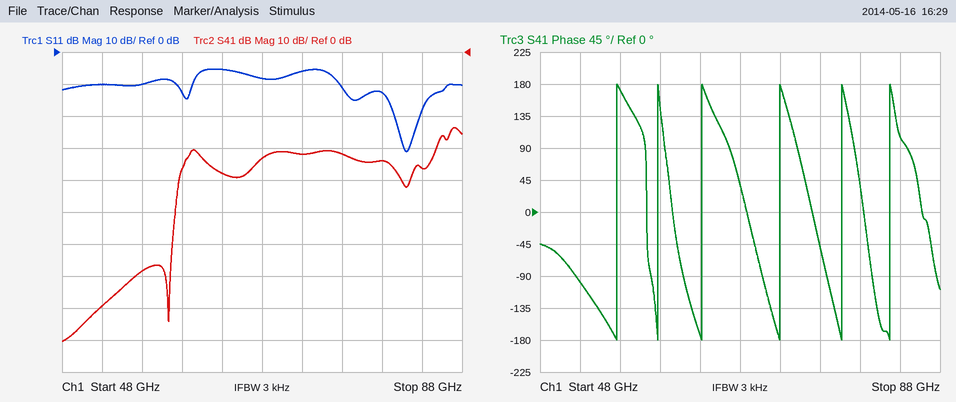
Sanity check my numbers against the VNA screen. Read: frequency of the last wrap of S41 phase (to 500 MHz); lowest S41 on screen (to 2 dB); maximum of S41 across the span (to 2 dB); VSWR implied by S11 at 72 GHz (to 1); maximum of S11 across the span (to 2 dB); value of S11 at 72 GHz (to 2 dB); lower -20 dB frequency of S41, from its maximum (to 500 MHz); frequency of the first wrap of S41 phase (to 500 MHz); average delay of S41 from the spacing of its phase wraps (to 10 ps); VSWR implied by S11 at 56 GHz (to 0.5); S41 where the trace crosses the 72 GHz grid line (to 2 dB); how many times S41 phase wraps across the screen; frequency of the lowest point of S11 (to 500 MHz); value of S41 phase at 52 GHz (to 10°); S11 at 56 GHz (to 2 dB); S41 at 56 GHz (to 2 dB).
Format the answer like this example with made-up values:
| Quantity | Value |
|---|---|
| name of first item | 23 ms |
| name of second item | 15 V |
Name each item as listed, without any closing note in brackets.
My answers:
| Quantity | Value |
|---|---|
| frequency of the last wrap of S41 phase | 83.0 GHz |
| lowest S41 on screen | -90 dB |
| maximum of S41 across the span | -24 dB |
| VSWR implied by S11 at 72 GHz | 3 |
| maximum of S11 across the span | -6 dB |
| value of S11 at 72 GHz | -6 dB |
| lower -20 dB frequency of S41, from its maximum | 59.5 GHz |
| frequency of the first wrap of S41 phase | 55.5 GHz |
| average delay of S41 from the spacing of its phase wraps | 180 ps |
| VSWR implied by S11 at 56 GHz | 2.0 |
| S41 where the trace crosses the 72 GHz grid line | -32 dB |
| how many times S41 phase wraps across the screen | 6 |
| frequency of the lowest point of S11 | 82.5 GHz |
| value of S41 phase at 52 GHz | -100° |
| S11 at 56 GHz | -10 dB |
| S41 at 56 GHz | -68 dB |
